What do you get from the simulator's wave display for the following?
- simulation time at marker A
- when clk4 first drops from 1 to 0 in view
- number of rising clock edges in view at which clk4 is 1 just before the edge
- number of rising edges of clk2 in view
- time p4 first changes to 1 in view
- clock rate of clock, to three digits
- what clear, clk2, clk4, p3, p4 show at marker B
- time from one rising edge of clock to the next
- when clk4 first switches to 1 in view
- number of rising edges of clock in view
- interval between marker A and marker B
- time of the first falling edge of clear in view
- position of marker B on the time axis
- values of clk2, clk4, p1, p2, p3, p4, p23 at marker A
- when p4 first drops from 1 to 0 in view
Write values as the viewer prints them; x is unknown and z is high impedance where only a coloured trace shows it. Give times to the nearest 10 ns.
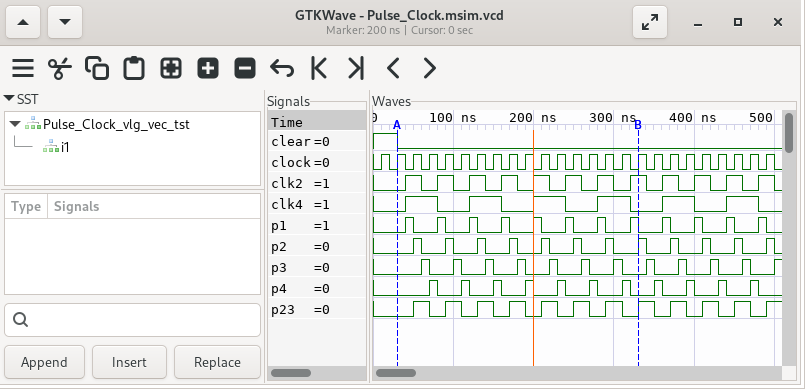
30 ns
80 ns
12
12
70 ns
50.0 MHz
clear=0, clk2=1, clk4=0, p3=0, p4=0
20 ns
40 ns
25
300 ns
30 ns
330 ns
clk2=0, clk4=0, p1=0, p2=0, p3=0, p4=0, p23=0
80 ns
